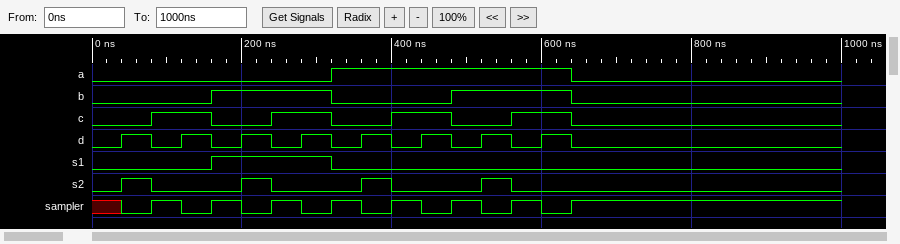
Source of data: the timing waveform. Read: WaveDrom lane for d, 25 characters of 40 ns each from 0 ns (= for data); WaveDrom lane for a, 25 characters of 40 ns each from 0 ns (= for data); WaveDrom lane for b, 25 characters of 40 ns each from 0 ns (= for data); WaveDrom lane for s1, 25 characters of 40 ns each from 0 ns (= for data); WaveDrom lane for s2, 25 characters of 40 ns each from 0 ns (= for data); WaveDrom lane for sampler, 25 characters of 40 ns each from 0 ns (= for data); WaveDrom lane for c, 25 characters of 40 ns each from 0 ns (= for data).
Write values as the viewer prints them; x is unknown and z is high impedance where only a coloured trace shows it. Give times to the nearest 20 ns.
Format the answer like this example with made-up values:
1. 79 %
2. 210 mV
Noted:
1. {name: 'd', wave: '01010101010101010........'}
2. {name: 'a', wave: '0.......1.......0........'}
3. {name: 'b', wave: '0...1...0...1...0........'}
4. {name: 's1', wave: '0...1...0................'}
5. {name: 's2', wave: '010..10..10..10..........'}
6. {name: 'sampler', wave: 'x0101010101010101........'}
7. {name: 'c', wave: '0.1.0.1.0.1.0.1.0........'}
